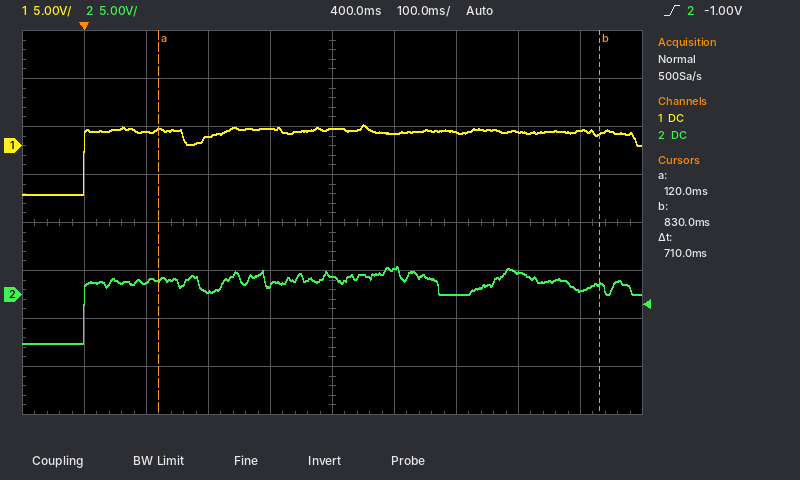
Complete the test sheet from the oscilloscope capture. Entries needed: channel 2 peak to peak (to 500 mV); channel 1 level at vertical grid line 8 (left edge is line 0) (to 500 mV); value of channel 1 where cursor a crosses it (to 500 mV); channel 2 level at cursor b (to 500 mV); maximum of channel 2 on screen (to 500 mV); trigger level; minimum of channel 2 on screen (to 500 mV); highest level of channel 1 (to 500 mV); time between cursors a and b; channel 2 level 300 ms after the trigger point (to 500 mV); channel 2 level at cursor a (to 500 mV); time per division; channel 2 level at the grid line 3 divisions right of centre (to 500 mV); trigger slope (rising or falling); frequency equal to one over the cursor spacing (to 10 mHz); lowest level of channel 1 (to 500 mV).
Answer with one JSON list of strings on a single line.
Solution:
["8.0 V", "1.5 V", "1.5 V", "1.0 V", "3.0 V", "-1.00 V", "-5.0 V", "2.0 V", "710 ms", "1.0 V", "1.5 V", "100 ms", "2.5 V", "rising", "1.41 Hz", "-5.0 V"]
